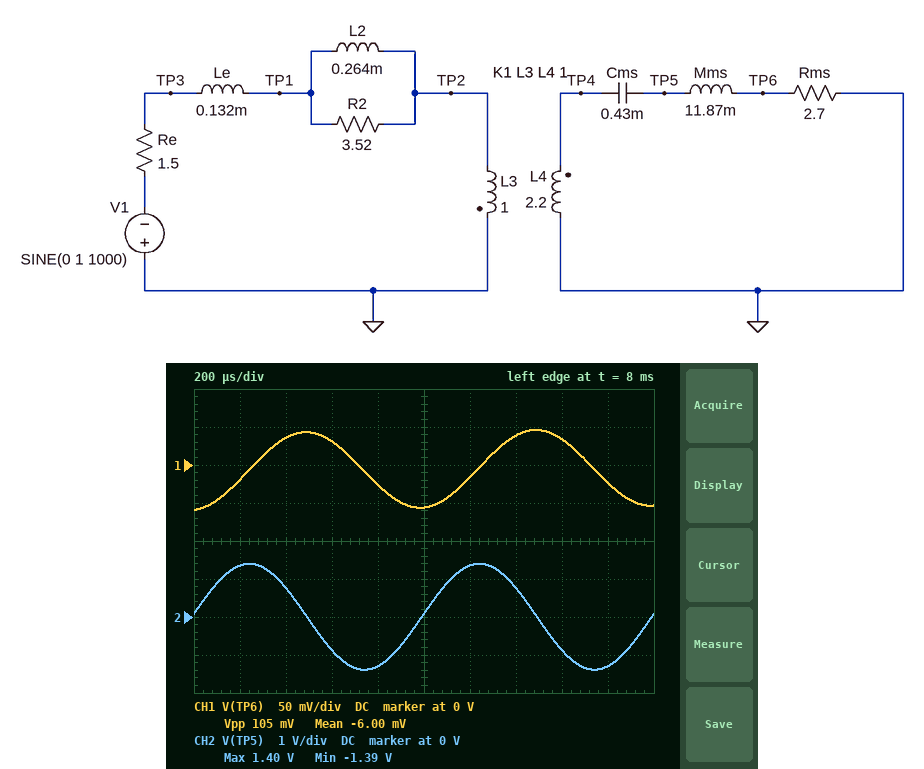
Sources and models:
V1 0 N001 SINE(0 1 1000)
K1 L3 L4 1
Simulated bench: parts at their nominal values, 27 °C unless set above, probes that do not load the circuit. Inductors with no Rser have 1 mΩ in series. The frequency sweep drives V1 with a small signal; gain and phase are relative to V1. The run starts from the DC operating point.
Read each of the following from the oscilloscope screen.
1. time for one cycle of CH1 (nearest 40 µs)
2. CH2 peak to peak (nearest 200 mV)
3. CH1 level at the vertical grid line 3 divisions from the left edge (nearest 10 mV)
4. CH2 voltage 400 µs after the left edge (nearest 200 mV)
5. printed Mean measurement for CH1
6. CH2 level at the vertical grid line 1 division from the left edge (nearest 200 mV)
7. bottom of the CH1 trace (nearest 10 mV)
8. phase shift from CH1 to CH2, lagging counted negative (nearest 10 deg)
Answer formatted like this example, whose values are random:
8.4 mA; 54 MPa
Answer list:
1.00 ms; 2.8 V; 30 mV; 800 mV; -6.00 mV; 1.4 V; -60 mV; 90 deg
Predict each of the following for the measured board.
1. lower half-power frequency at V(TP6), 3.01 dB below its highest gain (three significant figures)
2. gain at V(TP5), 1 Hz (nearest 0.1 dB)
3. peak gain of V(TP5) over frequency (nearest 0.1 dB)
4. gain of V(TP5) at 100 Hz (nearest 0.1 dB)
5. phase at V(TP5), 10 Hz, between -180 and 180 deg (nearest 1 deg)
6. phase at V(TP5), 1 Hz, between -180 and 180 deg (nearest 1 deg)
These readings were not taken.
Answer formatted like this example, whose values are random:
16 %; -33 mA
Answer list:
40.0 Hz; -39.5 dB; 4.0 dB; 4.0 dB; 97 deg; 104 deg
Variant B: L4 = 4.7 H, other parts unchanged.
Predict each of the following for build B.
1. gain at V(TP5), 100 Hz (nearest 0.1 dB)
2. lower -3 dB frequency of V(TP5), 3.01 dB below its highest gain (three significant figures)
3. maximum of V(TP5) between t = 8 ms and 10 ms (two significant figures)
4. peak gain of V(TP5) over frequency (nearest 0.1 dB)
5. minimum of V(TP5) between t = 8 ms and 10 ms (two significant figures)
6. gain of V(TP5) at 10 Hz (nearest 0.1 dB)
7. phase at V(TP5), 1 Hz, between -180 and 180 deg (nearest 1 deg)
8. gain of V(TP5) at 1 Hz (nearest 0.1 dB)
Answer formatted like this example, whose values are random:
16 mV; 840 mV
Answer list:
3.9 dB; 84.7 Hz; 1.9 V; 6.3 dB; -1.9 V; -15.8 dB; 104 deg; -36.2 dB
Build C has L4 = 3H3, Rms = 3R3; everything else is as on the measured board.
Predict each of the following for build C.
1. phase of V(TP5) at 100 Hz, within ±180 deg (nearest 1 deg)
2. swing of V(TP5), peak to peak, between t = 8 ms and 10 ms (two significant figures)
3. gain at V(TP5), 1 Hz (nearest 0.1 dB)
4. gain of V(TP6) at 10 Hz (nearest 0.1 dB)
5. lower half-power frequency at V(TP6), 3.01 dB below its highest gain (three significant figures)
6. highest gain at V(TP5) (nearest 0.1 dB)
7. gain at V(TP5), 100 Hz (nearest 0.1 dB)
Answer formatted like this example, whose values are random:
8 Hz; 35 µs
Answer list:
37 deg; 3.3 V; -36.0 dB; -15.8 dB; 33.4 Hz; 4.9 dB; 3.9 dB
